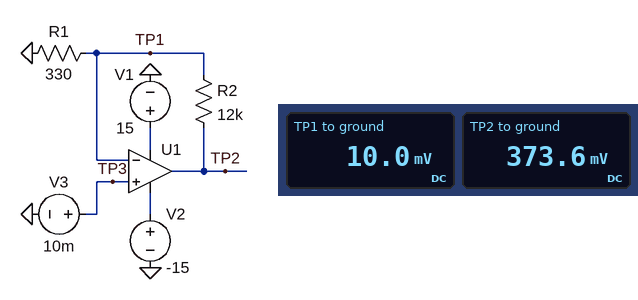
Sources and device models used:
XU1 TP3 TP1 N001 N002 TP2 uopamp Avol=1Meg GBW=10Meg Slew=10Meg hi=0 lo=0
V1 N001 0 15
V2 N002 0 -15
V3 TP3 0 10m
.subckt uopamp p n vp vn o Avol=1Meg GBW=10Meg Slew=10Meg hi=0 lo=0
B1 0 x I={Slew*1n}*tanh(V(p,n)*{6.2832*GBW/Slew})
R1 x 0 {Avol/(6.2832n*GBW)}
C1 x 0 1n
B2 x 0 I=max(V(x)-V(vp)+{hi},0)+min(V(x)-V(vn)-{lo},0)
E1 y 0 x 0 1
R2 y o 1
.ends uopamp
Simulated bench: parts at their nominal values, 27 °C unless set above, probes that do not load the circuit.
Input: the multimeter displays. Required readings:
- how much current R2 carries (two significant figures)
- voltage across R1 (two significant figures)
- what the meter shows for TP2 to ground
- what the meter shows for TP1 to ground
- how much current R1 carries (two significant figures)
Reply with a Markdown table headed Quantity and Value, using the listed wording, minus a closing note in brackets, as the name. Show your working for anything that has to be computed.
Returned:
| Quantity | Value |
|---|---|
| how much current R2 carries | (373.6 mV - 10 mV) / 12 kΩ = 30 µA |
| voltage across R1 | 10 mV = 10 mV |
| what the meter shows for TP2 to ground | 373.6 mV |
| what the meter shows for TP1 to ground | 10.0 mV |
| how much current R1 carries | (10 mV) / 330 Ω = 30 µA |
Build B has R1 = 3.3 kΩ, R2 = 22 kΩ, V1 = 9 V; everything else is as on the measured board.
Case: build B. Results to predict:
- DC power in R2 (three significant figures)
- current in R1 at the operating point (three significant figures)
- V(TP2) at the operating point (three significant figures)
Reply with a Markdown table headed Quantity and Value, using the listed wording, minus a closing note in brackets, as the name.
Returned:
| Quantity | Value |
|---|---|
| DC power in R2 | 202 nW |
| current in R1 at the operating point | 3.03 µA |
| V(TP2) at the operating point | 76.7 mV |
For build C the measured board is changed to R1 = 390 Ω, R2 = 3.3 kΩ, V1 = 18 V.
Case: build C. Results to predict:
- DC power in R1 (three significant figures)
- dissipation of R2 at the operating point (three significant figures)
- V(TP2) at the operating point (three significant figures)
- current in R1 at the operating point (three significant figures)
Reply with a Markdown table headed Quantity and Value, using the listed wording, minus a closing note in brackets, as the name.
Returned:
| Quantity | Value |
|---|---|
| DC power in R1 | 256 nW |
| dissipation of R2 at the operating point | 2.17 µW |
| V(TP2) at the operating point | 94.6 mV |
| current in R1 at the operating point | 25.6 µA |
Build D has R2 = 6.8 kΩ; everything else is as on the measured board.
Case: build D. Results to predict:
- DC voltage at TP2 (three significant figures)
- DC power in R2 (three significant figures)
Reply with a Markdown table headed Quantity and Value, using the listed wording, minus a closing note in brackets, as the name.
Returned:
| Quantity | Value |
|---|---|
| DC voltage at TP2 | 216 mV |
| DC power in R2 | 6.24 µW |
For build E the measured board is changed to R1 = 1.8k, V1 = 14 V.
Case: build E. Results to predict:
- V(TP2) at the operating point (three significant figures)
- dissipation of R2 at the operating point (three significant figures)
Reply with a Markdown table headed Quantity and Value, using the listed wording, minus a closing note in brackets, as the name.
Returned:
| Quantity | Value |
|---|---|
| V(TP2) at the operating point | 76.7 mV |
| dissipation of R2 at the operating point | 370 nW |
